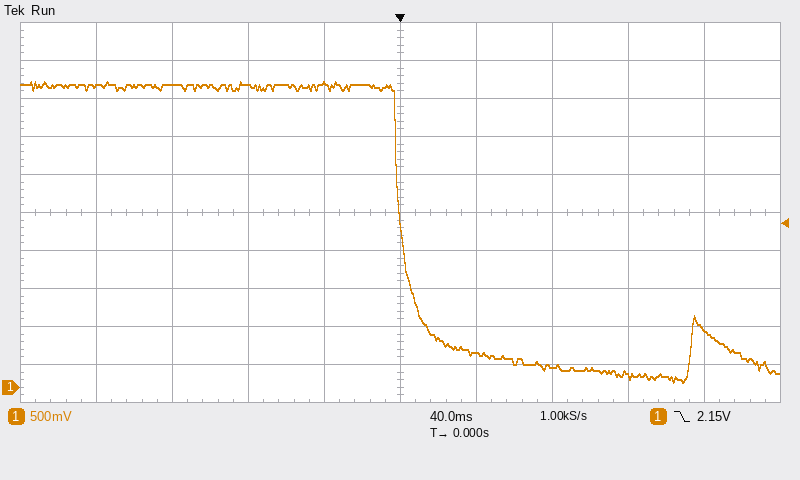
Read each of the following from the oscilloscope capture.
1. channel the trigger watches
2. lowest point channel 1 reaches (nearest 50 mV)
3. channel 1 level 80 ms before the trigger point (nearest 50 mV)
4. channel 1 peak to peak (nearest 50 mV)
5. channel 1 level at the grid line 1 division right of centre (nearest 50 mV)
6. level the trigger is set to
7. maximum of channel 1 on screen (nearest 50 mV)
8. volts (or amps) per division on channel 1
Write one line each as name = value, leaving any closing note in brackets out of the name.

channel the trigger watches = channel 1
lowest point channel 1 reaches = 50 mV
channel 1 level 80 ms before the trigger point = 3.95 V
channel 1 peak to peak = 3.95 V
channel 1 level at the grid line 1 division right of centre = 450 mV
level the trigger is set to = 2.15 V
maximum of channel 1 on screen = 4.00 V
volts (or amps) per division on channel 1 = 500 mV
